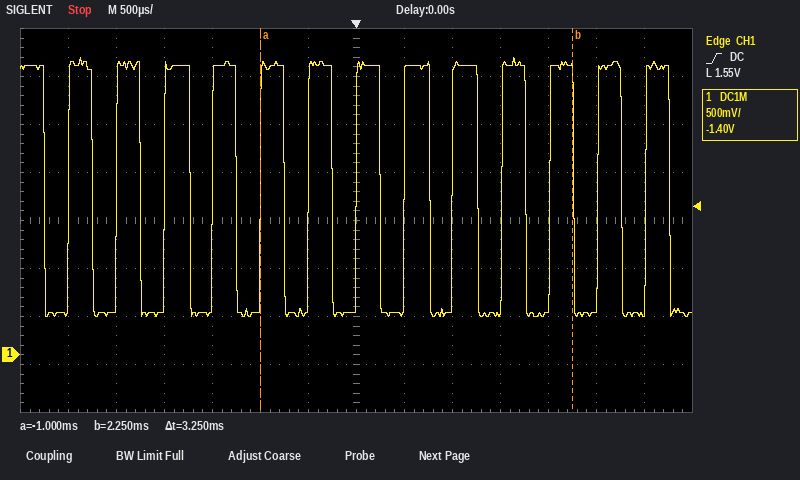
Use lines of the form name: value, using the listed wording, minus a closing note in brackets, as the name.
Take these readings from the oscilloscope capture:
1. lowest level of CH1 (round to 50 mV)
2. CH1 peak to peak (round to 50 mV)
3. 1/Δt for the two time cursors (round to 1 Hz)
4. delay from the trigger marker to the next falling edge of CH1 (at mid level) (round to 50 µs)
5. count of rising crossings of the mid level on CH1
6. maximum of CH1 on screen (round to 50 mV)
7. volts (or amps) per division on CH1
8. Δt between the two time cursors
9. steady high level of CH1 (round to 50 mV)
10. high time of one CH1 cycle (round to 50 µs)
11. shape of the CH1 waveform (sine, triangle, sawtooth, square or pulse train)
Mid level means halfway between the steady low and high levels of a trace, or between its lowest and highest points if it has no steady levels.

lowest level of CH1: 400 mV
CH1 peak to peak: 2.70 V
1/Δt for the two time cursors: 308 Hz
delay from the trigger marker to the next falling edge of CH1 (at mid level): 250 µs
count of rising crossings of the mid level on CH1: 13
maximum of CH1 on screen: 3.10 V
volts (or amps) per division on CH1: 500 mV
Δt between the two time cursors: 3.25 ms
steady high level of CH1: 3.00 V
high time of one CH1 cycle: 250 µs
shape of the CH1 waveform: square
